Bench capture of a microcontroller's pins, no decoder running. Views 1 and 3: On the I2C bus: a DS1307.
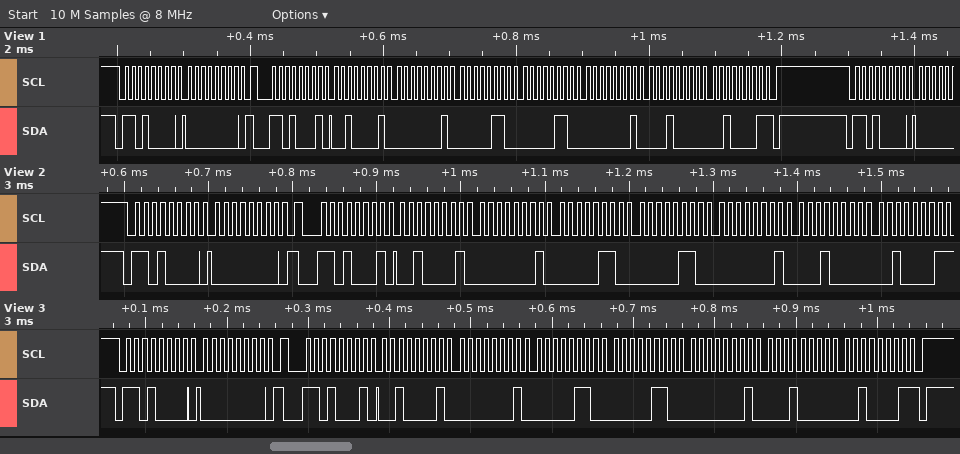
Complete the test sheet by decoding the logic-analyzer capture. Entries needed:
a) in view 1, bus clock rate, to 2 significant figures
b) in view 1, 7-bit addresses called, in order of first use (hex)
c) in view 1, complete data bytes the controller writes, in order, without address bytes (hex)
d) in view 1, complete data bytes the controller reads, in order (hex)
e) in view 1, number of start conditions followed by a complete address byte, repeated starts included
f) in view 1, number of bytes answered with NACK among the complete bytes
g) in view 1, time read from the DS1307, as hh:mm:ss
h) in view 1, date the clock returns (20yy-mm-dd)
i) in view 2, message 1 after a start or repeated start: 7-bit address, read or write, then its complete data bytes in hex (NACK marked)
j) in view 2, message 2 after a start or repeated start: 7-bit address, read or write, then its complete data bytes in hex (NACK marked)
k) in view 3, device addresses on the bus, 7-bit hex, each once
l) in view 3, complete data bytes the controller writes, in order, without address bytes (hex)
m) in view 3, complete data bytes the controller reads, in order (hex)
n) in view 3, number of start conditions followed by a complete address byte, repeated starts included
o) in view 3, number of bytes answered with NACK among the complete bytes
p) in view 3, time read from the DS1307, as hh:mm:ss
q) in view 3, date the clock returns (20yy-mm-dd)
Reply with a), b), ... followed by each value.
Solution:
a) 100 kHz
b) 0x68
c) 00
d) 21 01 06 06 01 10 21
e) 3
f) 1
g) 06:01:21
h) 2021-10-01
i) 0x68 write: 00
j) 0x68 read: 21 01 06 06 01 10 21 NACK
k) 0x68
l) 00
m) 21 01 06 06 01 10 21
n) 2
o) 1
p) 06:01:21
q) 2021-10-01
